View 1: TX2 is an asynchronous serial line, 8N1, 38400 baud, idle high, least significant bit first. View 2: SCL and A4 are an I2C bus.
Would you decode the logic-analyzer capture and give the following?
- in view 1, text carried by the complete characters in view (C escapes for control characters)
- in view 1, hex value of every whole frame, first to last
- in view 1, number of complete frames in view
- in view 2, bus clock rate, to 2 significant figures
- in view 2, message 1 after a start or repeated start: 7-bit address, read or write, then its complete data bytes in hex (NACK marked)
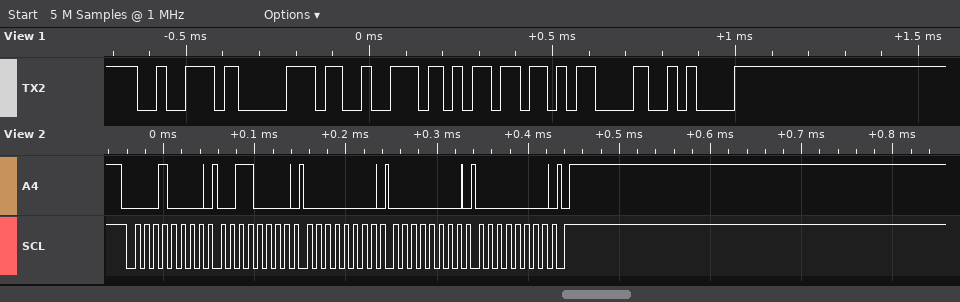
"rprm\r\n"
0x72 0x70 0x72 0x6D 0x0D 0x0A
6
100 kHz
0x08 write: 30 00 00 00
